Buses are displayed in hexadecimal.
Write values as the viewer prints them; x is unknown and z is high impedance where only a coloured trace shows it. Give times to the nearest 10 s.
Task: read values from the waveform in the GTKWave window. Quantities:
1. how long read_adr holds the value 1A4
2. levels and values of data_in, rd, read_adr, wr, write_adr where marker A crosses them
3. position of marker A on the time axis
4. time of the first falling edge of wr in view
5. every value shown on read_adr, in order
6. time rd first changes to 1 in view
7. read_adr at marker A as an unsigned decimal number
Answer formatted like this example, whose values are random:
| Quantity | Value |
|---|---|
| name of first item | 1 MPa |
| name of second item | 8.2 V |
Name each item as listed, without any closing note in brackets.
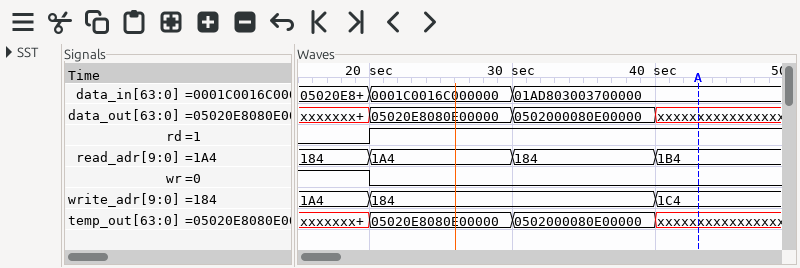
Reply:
| Quantity | Value |
|---|---|
| how long read_adr holds the value 1A4 | 10 s |
| levels and values of data_in, rd, read_adr, wr, write_adr where marker A crosses them | data_in=01AD803003700000, rd=1, read_adr=1B4, wr=0, write_adr=1C4 |
| position of marker A on the time axis | 40 s |
| time of the first falling edge of wr in view | 20 s |
| every value shown on read_adr, in order | 184, 1A4, 184, 1B4 |
| time rd first changes to 1 in view | 20 s |
| read_adr at marker A as an unsigned decimal number | 436 |
